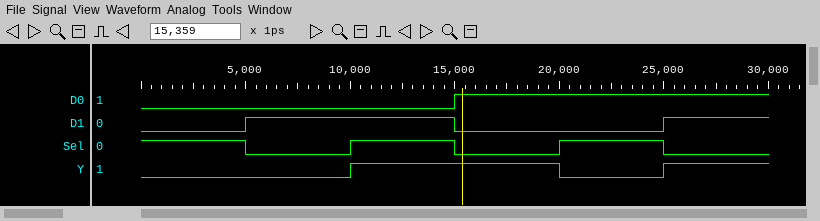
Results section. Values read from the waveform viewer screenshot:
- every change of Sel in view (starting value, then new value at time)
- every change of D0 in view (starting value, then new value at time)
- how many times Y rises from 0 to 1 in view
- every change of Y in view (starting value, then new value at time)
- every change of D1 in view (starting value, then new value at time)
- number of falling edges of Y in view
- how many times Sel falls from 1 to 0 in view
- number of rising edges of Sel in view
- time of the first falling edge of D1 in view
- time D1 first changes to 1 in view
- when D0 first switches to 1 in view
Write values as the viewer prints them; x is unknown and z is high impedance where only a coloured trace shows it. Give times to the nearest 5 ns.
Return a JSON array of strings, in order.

["1, 0 at 5 ns, 1 at 10 ns, 0 at 15 ns, 1 at 20 ns, 0 at 25 ns", "0, 1 at 15 ns", "2", "0, 1 at 10 ns, 0 at 20 ns, 1 at 25 ns", "0, 1 at 5 ns, 0 at 15 ns, 1 at 25 ns", "1", "3", "2", "15 ns", "5 ns", "15 ns"]
